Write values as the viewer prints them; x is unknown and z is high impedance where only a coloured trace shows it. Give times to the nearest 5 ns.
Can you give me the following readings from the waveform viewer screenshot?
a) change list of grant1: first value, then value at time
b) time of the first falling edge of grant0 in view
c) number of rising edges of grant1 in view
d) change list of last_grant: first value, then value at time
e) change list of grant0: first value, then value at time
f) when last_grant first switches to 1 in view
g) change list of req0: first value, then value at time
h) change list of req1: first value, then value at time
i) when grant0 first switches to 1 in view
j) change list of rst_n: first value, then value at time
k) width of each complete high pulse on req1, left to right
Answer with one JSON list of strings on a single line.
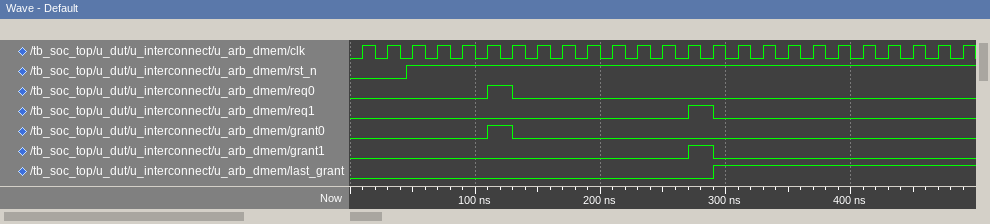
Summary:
["0, 1 at 270 ns, 0 at 290 ns", "130 ns", "1", "0, 1 at 290 ns", "0, 1 at 110 ns, 0 at 130 ns", "290 ns", "0, 1 at 110 ns, 0 at 130 ns", "0, 1 at 270 ns, 0 at 290 ns", "110 ns", "0, 1 at 45 ns", "20 ns"]
